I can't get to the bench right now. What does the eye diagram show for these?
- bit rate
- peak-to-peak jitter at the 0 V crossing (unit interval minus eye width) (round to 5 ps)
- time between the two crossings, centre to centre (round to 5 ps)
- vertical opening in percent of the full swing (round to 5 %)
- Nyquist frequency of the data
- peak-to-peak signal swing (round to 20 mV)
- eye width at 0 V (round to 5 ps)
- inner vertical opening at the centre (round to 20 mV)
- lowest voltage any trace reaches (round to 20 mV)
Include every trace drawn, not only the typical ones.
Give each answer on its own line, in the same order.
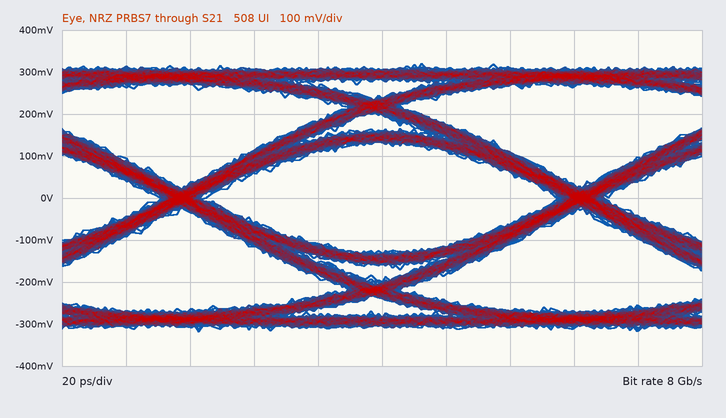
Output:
8 Gb/s
15 ps
125 ps
40 %
4 GHz
640 mV
110 ps
260 mV
-320 mV
